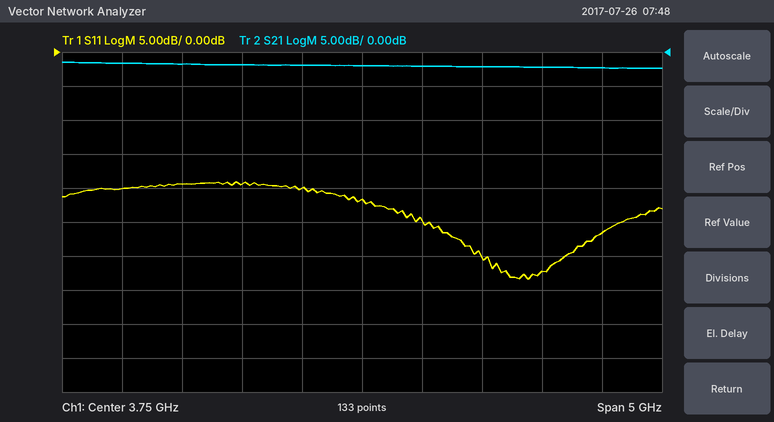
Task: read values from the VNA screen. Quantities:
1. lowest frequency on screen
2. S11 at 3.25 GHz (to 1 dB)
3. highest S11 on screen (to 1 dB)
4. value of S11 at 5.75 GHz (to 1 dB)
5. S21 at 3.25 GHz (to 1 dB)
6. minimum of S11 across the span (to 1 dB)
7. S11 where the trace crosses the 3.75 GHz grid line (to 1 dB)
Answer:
1.25 GHz
-20 dB
-19 dB
-27 dB
-2 dB
-33 dB
-22 dB
